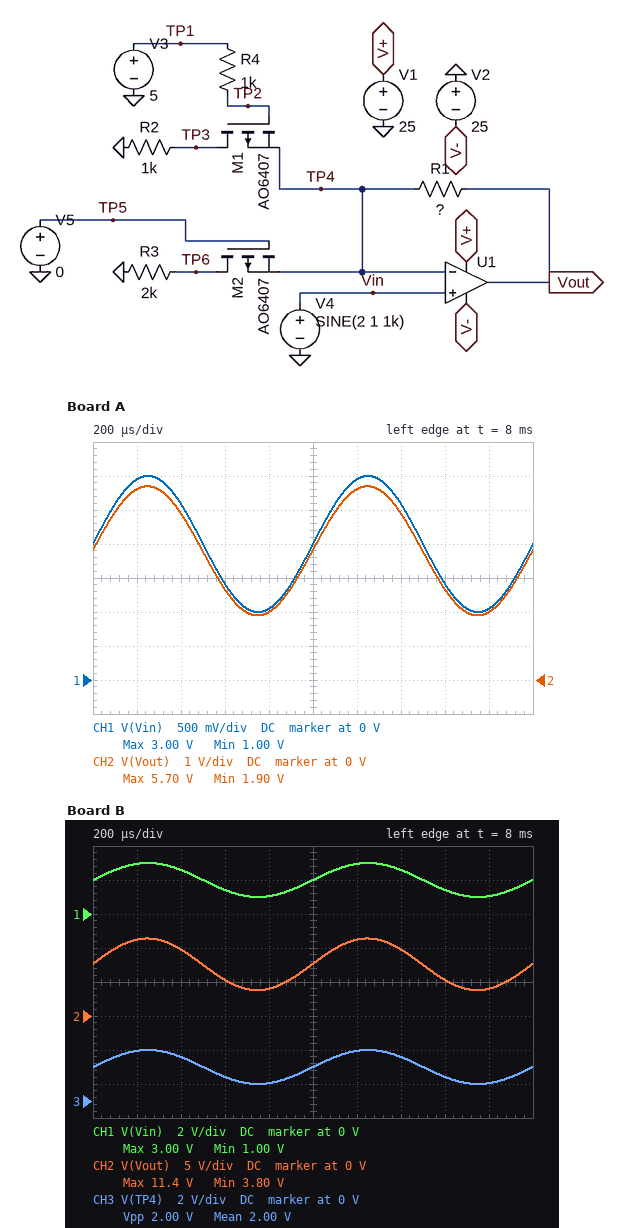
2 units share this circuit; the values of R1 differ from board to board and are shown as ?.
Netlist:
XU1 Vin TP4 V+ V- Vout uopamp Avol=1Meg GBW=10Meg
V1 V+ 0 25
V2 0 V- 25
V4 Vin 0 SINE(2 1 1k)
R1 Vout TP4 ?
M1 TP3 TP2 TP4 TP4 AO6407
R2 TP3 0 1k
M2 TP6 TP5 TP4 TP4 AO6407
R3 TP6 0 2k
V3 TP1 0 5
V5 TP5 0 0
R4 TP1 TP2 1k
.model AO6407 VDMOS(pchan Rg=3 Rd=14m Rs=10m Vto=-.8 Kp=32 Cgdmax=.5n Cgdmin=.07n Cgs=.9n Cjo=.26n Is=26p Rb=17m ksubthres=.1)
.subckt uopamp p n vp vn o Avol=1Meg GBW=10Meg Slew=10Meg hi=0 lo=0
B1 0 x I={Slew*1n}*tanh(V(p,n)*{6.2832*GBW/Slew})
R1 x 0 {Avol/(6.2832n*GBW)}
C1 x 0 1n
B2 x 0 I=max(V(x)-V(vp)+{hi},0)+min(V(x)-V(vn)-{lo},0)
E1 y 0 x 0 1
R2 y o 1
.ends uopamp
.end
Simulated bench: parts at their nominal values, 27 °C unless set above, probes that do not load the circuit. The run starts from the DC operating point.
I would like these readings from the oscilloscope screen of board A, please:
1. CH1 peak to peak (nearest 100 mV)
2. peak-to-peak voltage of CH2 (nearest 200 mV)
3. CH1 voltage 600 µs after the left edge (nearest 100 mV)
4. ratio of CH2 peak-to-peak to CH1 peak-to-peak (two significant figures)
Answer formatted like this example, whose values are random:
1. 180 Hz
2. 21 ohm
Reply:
1. 2.0 V
2. 3.8 V
3. 1.4 V
4. 1.9
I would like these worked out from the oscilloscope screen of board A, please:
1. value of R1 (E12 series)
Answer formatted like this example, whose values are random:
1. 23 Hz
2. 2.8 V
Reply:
1. 1.8 kΩ
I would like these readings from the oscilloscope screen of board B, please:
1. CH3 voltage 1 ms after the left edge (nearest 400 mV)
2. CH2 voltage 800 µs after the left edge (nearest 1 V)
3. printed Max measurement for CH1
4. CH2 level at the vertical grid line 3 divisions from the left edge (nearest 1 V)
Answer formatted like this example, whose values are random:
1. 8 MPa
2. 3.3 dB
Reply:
1. 2.0 V
2. 4 V
3. 3.00 V
4. 5 V
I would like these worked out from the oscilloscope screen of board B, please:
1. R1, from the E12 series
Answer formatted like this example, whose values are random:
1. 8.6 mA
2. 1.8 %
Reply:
1. 5.6 kΩ
